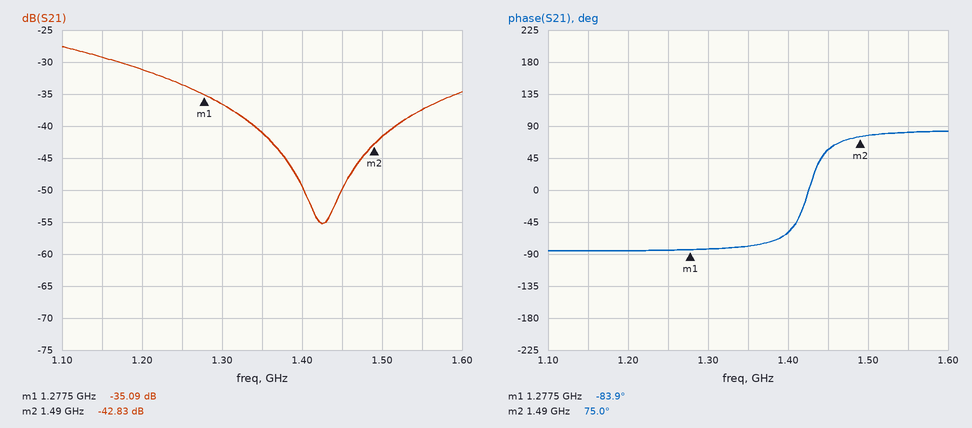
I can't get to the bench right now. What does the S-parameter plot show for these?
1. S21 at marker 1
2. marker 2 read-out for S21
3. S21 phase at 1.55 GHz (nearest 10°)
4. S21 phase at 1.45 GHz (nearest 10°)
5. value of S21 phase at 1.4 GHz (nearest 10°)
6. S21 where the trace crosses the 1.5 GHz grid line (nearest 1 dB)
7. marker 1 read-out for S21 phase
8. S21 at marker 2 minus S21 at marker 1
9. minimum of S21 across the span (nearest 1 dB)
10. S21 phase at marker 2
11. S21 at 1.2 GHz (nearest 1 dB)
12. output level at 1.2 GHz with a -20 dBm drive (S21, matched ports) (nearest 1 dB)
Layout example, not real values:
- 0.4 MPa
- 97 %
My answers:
- -35.09 dB
- -42.83 dB
- 80°
- 60°
- -60°
- -42 dB
- -83.9°
- -7.74 dB
- -55 dB
- 75.0°
- -31 dB
- -51 dBm
